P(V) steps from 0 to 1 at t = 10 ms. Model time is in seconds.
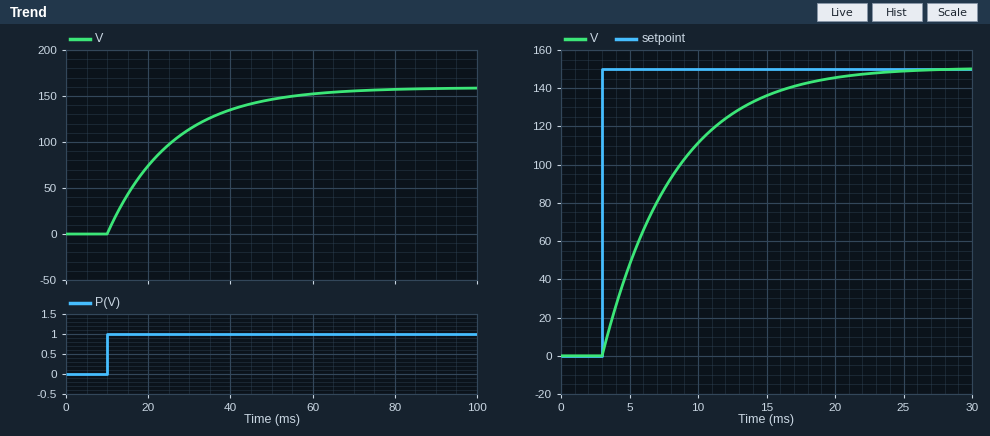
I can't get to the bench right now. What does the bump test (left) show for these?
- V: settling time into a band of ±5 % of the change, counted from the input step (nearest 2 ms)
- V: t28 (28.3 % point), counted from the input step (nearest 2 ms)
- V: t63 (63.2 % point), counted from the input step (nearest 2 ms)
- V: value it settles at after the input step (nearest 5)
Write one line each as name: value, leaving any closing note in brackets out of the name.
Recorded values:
V: settling time into a band of ±5 % of the change, counted from the input step: 48 ms
V: t28 (28.3 % point), counted from the input step: 6 ms
V: t63 (63.2 % point), counted from the input step: 16 ms
V: value it settles at after the input step: 160
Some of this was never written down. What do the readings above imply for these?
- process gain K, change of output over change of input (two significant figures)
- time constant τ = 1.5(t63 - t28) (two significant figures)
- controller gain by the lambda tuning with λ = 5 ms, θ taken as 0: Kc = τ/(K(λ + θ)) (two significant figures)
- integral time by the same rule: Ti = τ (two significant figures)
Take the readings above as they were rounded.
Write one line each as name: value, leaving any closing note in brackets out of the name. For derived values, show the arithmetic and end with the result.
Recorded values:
process gain K, change of output over change of input: (160 - 0) / 1 = 160
time constant τ = 1.5(t63 - t28): 1.5 × (16 - 6) = 15 ms
controller gain by the lambda tuning with λ = 5 ms, θ taken as 0: Kc = τ/(K(λ + θ)): 15 / (160 × (5 + 0)) = 0.019
integral time by the same rule: Ti = τ: 15 ms
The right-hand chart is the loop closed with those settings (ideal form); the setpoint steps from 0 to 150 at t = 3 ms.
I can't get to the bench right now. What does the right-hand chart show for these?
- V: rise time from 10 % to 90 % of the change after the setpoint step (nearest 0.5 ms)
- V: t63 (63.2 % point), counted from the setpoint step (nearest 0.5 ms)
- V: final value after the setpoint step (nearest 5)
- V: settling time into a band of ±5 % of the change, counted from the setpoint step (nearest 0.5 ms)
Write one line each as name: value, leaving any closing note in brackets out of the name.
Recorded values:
V: rise time from 10 % to 90 % of the change after the setpoint step: 11.0 ms
V: t63 (63.2 % point), counted from the setpoint step: 5.0 ms
V: final value after the setpoint step: 150
V: settling time into a band of ±5 % of the change, counted from the setpoint step: 15.0 ms
